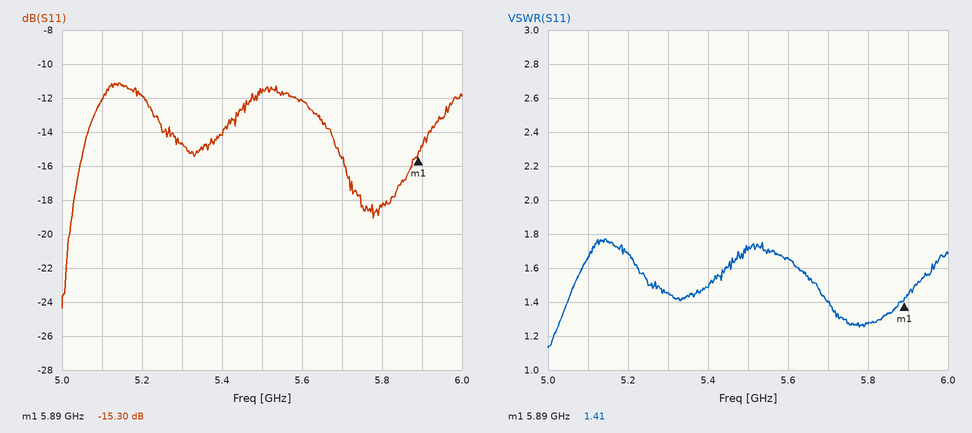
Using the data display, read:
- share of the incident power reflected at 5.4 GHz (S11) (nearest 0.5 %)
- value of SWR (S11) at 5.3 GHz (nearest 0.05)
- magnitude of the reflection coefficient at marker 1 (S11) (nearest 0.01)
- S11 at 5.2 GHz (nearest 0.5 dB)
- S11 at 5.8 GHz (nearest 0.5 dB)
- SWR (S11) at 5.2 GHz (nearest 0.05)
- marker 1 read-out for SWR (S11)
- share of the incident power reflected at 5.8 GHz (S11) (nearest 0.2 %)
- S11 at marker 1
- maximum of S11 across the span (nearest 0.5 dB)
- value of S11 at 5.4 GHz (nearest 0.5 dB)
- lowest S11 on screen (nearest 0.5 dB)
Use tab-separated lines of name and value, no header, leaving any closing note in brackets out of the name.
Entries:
share of the incident power reflected at 5.4 GHz (S11)	4.0 %
value of SWR (S11) at 5.3 GHz	1.45
magnitude of the reflection coefficient at marker 1 (S11)	0.17
S11 at 5.2 GHz	-12.0 dB
S11 at 5.8 GHz	-18.5 dB
SWR (S11) at 5.2 GHz	1.70
marker 1 read-out for SWR	1.41
share of the incident power reflected at 5.8 GHz (S11)	1.4 %
S11 at marker 1	-15.30 dB
maximum of S11 across the span	-11.0 dB
value of S11 at 5.4 GHz	-14.0 dB
lowest S11 on screen	-24.5 dB
